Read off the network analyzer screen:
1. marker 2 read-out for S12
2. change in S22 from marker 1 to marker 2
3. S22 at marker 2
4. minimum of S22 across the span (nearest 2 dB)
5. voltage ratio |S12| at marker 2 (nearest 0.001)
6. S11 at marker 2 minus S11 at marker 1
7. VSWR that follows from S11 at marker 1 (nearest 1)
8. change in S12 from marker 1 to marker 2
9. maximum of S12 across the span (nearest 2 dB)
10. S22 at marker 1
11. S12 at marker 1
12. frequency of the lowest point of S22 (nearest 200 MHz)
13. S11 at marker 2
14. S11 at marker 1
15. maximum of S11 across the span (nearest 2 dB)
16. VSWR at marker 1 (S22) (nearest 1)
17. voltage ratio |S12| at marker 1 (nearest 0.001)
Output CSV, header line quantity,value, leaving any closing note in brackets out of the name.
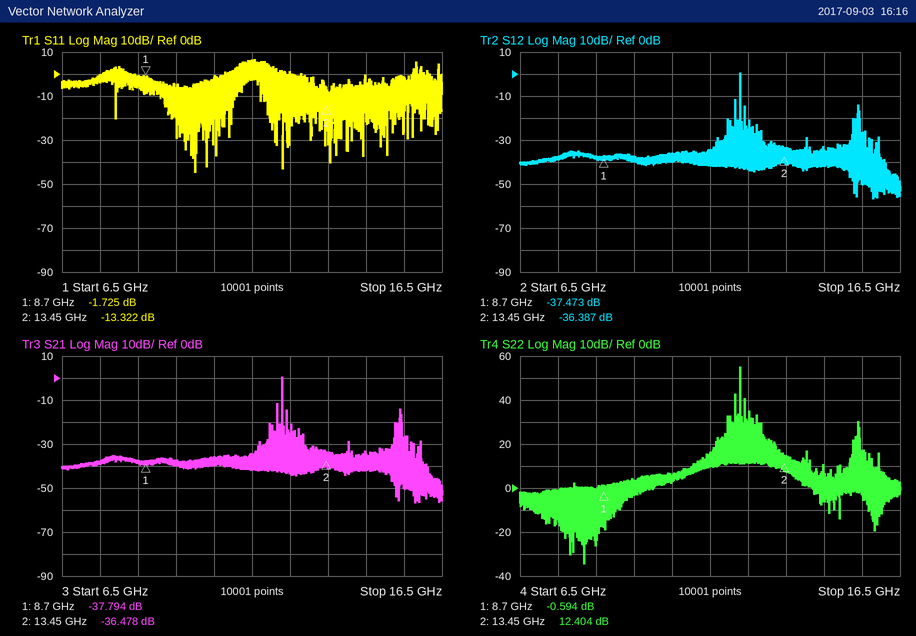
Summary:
quantity,value
marker 2 read-out for S12,-36.387 dB
change in S22 from marker 1 to marker 2,12.998 dB
S22 at marker 2,12.404 dB
minimum of S22 across the span,-34 dB
voltage ratio |S12| at marker 2,0.015
S11 at marker 2 minus S11 at marker 1,-11.597 dB
VSWR that follows from S11 at marker 1,10
change in S12 from marker 1 to marker 2,1.086 dB
maximum of S12 across the span,0 dB
S22 at marker 1,-0.594 dB
S12 at marker 1,-37.473 dB
frequency of the lowest point of S22,8.2 GHz
S11 at marker 2,-13.322 dB
S11 at marker 1,-1.725 dB
maximum of S11 across the span,6 dB
VSWR at marker 1 (S22),29
voltage ratio |S12| at marker 1,0.013
